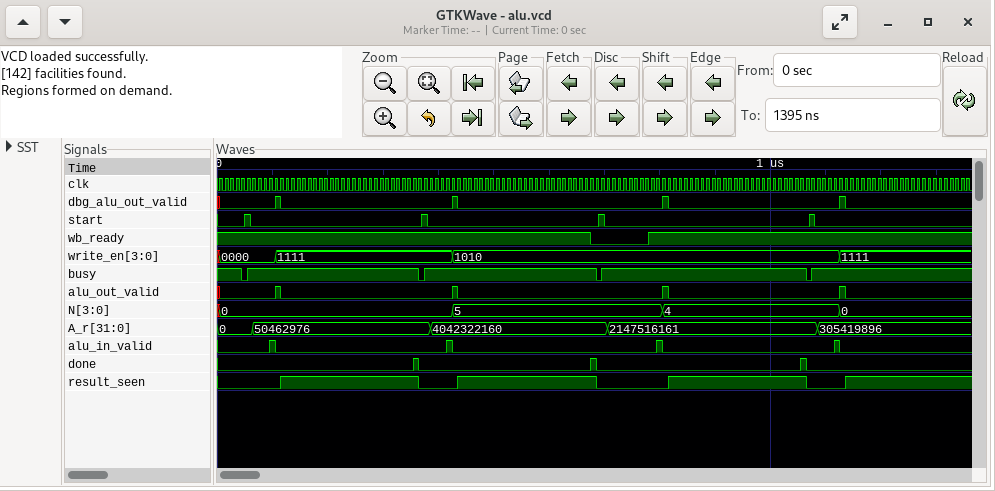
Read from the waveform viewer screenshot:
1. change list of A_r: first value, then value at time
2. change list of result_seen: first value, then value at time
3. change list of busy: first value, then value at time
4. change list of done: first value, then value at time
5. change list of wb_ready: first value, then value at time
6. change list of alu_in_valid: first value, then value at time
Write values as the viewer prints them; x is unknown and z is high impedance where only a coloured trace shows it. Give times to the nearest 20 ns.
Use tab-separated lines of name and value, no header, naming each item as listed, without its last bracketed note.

change list of A_r: first value, then value at time	0, 50462976 at 60 ns, 4042322160 at 380 ns, 2147516161 at 700 ns, 305419896 at 1080 ns
change list of result_seen: first value, then value at time	0, 1 at 120 ns, 0 at 360 ns, 1 at 440 ns, 0 at 680 ns, 1 at 820 ns, 0 at 1060 ns, 1 at 1140 ns
change list of busy: first value, then value at time	1, 0 at 40 ns, 1 at 60 ns, 0 at 360 ns, 1 at 380 ns, 0 at 680 ns, 1 at 700 ns, 0 at 1060 ns, 1 at 1080 ns
change list of done: first value, then value at time	0, 1 at 360 ns, 0 at 360 ns, 1 at 680 ns, 0 at 680 ns, 1 at 1060 ns, 0 at 1060 ns
change list of wb_ready: first value, then value at time	1, 0 at 680 ns, 1 at 780 ns
change list of alu_in_valid: first value, then value at time	0, 1 at 100 ns, 0 at 100 ns, 1 at 420 ns, 0 at 420 ns, 1 at 800 ns, 0 at 800 ns, 1 at 1120 ns, 0 at 1120 ns
